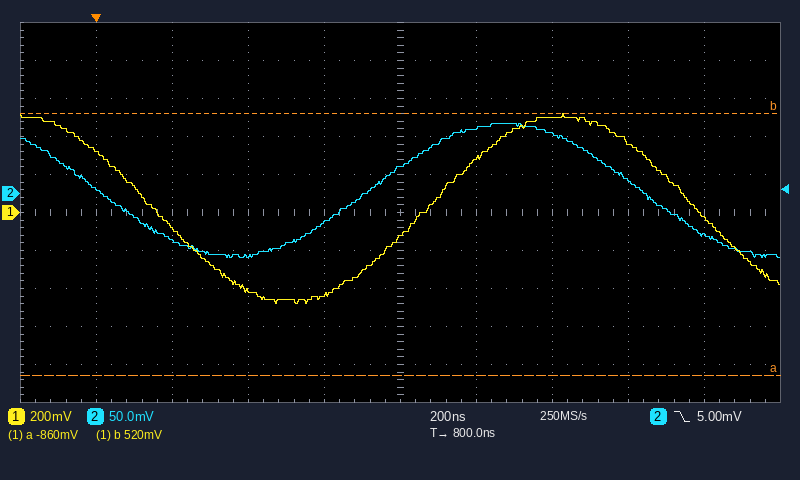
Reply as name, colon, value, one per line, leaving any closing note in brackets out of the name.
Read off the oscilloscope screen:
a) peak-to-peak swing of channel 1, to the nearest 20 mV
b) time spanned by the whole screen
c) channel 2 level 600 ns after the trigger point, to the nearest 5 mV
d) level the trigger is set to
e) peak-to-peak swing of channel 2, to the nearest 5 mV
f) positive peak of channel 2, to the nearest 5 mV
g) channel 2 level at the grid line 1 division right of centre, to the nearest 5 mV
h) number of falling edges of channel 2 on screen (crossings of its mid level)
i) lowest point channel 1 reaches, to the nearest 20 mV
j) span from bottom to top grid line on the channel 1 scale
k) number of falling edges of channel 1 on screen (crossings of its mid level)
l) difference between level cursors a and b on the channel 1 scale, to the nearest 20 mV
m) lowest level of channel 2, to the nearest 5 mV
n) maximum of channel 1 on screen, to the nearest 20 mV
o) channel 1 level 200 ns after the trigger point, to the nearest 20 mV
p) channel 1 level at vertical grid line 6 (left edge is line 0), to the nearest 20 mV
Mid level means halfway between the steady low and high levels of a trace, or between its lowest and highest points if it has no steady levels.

peak-to-peak swing of channel 1, to the nearest 20 mV: 1.00 V
time spanned by the whole screen: 2 µs
channel 2 level 600 ns after the trigger point, to the nearest 5 mV: -40 mV
level the trigger is set to: 5.00 mV
peak-to-peak swing of channel 2, to the nearest 5 mV: 175 mV
positive peak of channel 2, to the nearest 5 mV: 90 mV
channel 2 level at the grid line 1 division right of centre, to the nearest 5 mV: 85 mV
number of falling edges of channel 2 on screen: 2
lowest point channel 1 reaches, to the nearest 20 mV: -480 mV
span from bottom to top grid line on the channel 1 scale: 2 V
number of falling edges of channel 1 on screen: 2
difference between level cursors a and b on the channel 1 scale, to the nearest 20 mV: 1.38 V
lowest level of channel 2, to the nearest 5 mV: -85 mV
maximum of channel 1 on screen, to the nearest 20 mV: 520 mV
channel 1 level 200 ns after the trigger point, to the nearest 20 mV: -80 mV
channel 1 level at vertical grid line 6 (left edge is line 0), to the nearest 20 mV: 280 mV
